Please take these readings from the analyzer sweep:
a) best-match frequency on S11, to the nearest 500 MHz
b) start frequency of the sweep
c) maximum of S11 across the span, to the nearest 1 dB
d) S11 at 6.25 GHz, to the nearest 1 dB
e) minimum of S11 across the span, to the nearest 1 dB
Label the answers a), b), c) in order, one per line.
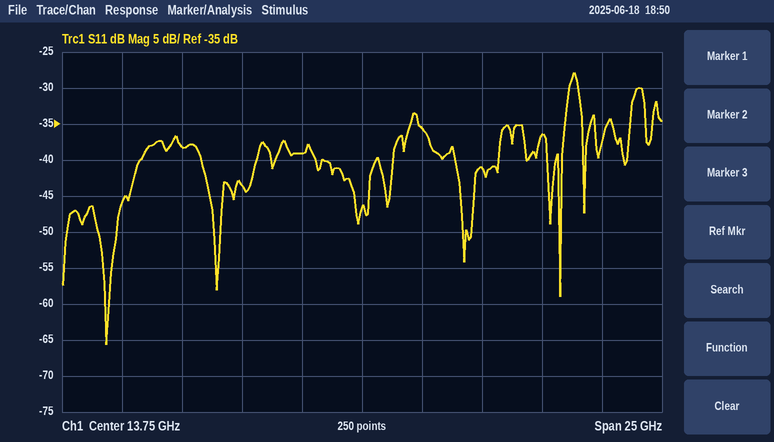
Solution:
a) 3.0 GHz
b) 1.25 GHz
c) -28 dB
d) -38 dB
e) -66 dB
